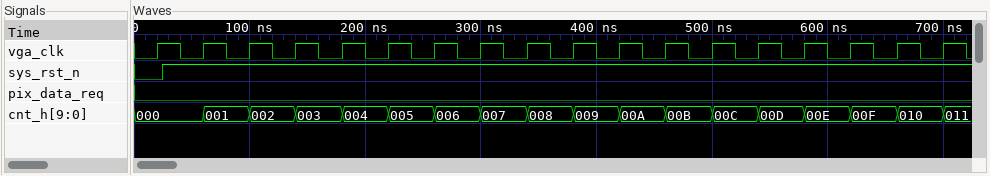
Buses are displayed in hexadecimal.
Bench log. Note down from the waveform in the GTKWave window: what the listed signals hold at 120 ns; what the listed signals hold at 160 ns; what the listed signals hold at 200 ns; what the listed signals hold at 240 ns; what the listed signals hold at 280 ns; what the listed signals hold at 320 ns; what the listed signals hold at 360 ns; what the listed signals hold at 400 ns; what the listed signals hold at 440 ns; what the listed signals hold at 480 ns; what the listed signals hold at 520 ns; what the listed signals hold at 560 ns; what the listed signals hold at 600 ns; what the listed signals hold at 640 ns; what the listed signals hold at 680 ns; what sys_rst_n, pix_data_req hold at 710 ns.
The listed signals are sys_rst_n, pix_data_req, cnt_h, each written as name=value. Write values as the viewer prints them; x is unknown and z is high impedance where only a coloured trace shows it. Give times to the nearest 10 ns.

sys_rst_n=1, pix_data_req=0, cnt_h=002
sys_rst_n=1, pix_data_req=0, cnt_h=003
sys_rst_n=1, pix_data_req=0, cnt_h=004
sys_rst_n=1, pix_data_req=0, cnt_h=005
sys_rst_n=1, pix_data_req=0, cnt_h=006
sys_rst_n=1, pix_data_req=0, cnt_h=007
sys_rst_n=1, pix_data_req=0, cnt_h=008
sys_rst_n=1, pix_data_req=0, cnt_h=009
sys_rst_n=1, pix_data_req=0, cnt_h=00A
sys_rst_n=1, pix_data_req=0, cnt_h=00B
sys_rst_n=1, pix_data_req=0, cnt_h=00C
sys_rst_n=1, pix_data_req=0, cnt_h=00D
sys_rst_n=1, pix_data_req=0, cnt_h=00E
sys_rst_n=1, pix_data_req=0, cnt_h=00F
sys_rst_n=1, pix_data_req=0, cnt_h=010
sys_rst_n=1, pix_data_req=0
